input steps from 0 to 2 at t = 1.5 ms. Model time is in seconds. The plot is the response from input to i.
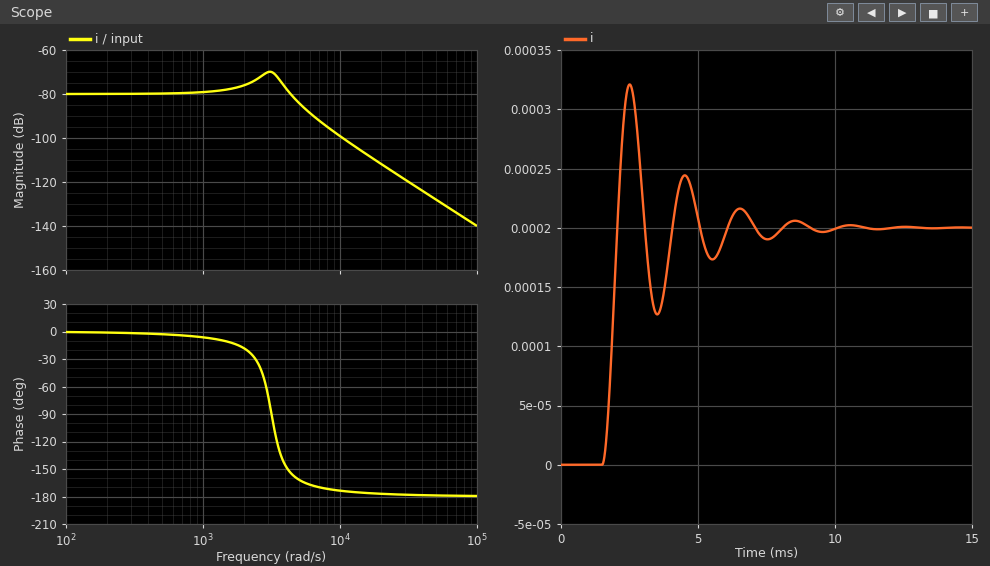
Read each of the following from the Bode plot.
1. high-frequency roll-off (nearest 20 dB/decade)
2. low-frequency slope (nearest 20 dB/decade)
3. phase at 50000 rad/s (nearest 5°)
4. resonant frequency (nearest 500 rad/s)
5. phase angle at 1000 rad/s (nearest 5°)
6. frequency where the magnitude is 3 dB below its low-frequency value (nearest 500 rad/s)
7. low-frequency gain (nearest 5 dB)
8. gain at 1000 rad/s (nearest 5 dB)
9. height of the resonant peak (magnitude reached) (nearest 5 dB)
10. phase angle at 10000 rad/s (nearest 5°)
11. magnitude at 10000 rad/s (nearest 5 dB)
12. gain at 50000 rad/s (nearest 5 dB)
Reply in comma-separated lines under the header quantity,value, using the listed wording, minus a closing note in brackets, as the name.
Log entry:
quantity,value
high-frequency roll-off,-40 dB/decade
low-frequency slope,0 dB/decade
phase at 50000 rad/s,-180°
resonant frequency,3000 rad/s
phase angle at 1000 rad/s,-5°
frequency where the magnitude is 3 dB below its low-frequency value,5000 rad/s
low-frequency gain,-80 dB
gain at 1000 rad/s,-80 dB
height of the resonant peak (magnitude reached),-70 dB
phase angle at 10000 rad/s,-175°
magnitude at 10000 rad/s,-100 dB
gain at 50000 rad/s,-130 dB
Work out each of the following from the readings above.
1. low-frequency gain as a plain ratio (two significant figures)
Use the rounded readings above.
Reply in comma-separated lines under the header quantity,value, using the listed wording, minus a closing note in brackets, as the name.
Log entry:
quantity,value
low-frequency gain as a plain ratio,0.00010
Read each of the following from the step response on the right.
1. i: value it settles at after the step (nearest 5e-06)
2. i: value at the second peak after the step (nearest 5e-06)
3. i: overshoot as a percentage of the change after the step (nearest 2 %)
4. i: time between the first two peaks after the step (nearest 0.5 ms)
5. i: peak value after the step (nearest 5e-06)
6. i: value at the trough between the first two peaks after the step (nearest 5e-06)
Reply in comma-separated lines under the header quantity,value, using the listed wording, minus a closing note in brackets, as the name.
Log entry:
quantity,value
i: value it settles at after the step,0.000200
i: value at the second peak after the step,0.000245
i: overshoot as a percentage of the change after the step,60 %
i: time between the first two peaks after the step,2.0 ms
i: peak value after the step,0.000320
i: value at the trough between the first two peaks after the step,0.000125
